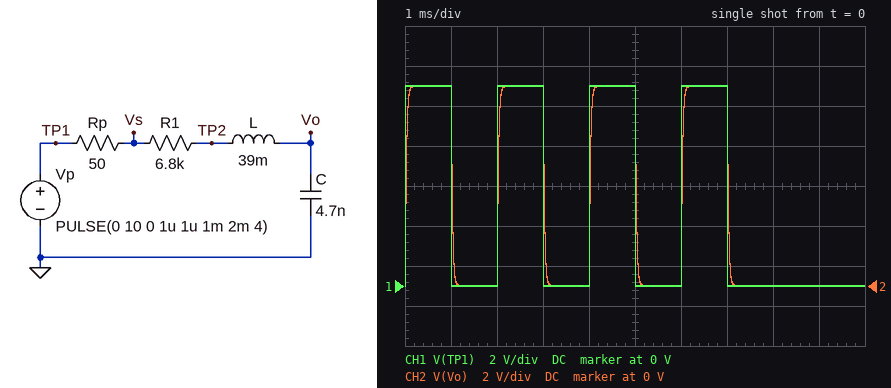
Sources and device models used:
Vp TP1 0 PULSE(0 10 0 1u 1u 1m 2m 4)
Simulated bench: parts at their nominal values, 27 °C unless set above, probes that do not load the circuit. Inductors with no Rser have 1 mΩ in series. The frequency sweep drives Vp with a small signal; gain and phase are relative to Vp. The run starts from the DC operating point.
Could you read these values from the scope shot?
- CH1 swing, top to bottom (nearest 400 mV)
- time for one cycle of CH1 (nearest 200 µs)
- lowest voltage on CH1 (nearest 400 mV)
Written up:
10.0 V
2.0 ms
0 V
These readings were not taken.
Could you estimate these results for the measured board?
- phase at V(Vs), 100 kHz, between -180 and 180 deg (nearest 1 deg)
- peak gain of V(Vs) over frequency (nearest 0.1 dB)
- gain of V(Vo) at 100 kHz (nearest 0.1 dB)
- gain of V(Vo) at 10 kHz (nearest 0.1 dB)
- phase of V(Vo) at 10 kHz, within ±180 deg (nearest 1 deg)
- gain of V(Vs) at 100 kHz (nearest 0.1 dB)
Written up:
0 deg
0 dB
-37.4 dB
-6.2 dB
-82 deg
0 dB
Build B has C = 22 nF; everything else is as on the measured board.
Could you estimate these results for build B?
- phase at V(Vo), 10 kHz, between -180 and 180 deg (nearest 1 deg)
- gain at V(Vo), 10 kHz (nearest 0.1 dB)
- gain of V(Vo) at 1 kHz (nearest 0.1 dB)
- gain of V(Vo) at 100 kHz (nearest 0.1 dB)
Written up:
-104 deg
-19.8 dB
-2.6 dB
-50.9 dB
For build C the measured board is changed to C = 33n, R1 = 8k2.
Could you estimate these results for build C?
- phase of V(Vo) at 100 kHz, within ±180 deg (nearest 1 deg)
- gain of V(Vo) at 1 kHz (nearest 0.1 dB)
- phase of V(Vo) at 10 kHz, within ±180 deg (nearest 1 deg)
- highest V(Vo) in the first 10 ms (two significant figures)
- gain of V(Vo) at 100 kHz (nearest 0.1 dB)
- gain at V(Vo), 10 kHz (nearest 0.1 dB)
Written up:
-161 deg
-5.8 dB
-103 deg
9.8 V
-54.6 dB
-24.9 dB
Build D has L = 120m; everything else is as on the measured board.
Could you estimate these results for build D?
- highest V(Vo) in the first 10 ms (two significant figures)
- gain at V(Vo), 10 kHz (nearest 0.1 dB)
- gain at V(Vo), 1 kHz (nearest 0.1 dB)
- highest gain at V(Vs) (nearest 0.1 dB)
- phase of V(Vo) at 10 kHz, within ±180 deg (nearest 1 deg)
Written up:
11 V
-7.5 dB
0 dB
0 dB
-121 deg
